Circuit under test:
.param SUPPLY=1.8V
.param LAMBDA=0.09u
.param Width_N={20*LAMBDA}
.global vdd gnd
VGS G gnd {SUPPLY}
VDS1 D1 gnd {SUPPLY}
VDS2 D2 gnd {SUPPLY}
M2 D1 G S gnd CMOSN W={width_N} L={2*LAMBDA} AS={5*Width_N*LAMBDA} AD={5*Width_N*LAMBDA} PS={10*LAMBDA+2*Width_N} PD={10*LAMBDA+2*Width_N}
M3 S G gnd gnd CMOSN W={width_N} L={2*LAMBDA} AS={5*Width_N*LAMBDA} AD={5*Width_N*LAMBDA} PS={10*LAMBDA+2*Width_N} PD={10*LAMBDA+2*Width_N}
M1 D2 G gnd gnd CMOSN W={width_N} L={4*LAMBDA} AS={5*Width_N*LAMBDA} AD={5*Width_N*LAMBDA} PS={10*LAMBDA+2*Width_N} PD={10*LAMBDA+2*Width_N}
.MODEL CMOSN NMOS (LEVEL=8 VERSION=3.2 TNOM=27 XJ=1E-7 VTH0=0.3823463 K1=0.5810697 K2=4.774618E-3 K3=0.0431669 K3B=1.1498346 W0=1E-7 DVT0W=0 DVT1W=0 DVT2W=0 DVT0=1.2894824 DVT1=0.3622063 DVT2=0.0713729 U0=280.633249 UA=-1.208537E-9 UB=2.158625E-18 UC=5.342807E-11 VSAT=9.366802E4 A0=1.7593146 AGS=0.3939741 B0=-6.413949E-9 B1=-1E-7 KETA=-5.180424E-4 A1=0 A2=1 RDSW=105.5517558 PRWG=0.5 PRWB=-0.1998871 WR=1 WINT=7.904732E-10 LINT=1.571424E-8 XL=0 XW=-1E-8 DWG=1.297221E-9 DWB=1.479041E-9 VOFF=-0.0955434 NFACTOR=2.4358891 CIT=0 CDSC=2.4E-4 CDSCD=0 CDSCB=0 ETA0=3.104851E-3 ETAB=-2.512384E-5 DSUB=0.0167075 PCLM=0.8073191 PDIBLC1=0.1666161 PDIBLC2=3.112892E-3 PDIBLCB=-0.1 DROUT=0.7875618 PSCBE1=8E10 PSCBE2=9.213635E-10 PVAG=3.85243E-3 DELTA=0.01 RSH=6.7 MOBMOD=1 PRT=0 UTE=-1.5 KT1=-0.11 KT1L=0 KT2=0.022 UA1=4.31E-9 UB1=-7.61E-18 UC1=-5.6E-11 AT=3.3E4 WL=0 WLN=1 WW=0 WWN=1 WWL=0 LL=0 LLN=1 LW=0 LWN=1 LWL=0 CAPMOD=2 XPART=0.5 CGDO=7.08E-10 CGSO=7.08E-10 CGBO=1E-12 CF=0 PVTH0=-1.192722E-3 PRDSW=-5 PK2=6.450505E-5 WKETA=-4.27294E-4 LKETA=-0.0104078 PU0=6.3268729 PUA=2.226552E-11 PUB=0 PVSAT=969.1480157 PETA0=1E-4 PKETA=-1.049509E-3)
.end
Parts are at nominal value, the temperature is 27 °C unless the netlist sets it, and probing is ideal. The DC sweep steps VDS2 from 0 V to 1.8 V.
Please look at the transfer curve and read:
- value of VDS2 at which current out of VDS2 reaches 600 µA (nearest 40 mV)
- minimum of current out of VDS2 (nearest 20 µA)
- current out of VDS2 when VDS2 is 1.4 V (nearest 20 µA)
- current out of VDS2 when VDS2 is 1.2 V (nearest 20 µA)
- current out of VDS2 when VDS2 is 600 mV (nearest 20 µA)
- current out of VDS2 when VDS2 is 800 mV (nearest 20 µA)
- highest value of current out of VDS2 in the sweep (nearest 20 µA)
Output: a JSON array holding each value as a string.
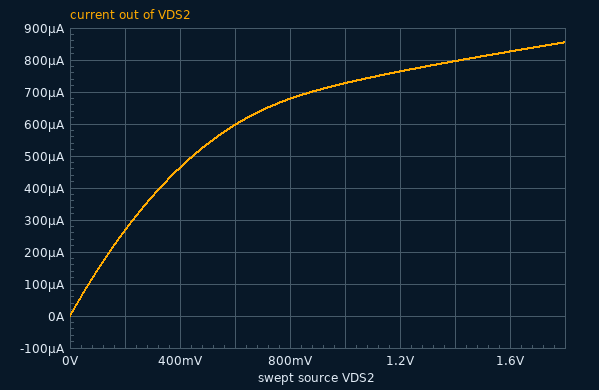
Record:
["600 mV", "0 A", "800 µA", "760 µA", "600 µA", "680 µA", "860 µA"]
